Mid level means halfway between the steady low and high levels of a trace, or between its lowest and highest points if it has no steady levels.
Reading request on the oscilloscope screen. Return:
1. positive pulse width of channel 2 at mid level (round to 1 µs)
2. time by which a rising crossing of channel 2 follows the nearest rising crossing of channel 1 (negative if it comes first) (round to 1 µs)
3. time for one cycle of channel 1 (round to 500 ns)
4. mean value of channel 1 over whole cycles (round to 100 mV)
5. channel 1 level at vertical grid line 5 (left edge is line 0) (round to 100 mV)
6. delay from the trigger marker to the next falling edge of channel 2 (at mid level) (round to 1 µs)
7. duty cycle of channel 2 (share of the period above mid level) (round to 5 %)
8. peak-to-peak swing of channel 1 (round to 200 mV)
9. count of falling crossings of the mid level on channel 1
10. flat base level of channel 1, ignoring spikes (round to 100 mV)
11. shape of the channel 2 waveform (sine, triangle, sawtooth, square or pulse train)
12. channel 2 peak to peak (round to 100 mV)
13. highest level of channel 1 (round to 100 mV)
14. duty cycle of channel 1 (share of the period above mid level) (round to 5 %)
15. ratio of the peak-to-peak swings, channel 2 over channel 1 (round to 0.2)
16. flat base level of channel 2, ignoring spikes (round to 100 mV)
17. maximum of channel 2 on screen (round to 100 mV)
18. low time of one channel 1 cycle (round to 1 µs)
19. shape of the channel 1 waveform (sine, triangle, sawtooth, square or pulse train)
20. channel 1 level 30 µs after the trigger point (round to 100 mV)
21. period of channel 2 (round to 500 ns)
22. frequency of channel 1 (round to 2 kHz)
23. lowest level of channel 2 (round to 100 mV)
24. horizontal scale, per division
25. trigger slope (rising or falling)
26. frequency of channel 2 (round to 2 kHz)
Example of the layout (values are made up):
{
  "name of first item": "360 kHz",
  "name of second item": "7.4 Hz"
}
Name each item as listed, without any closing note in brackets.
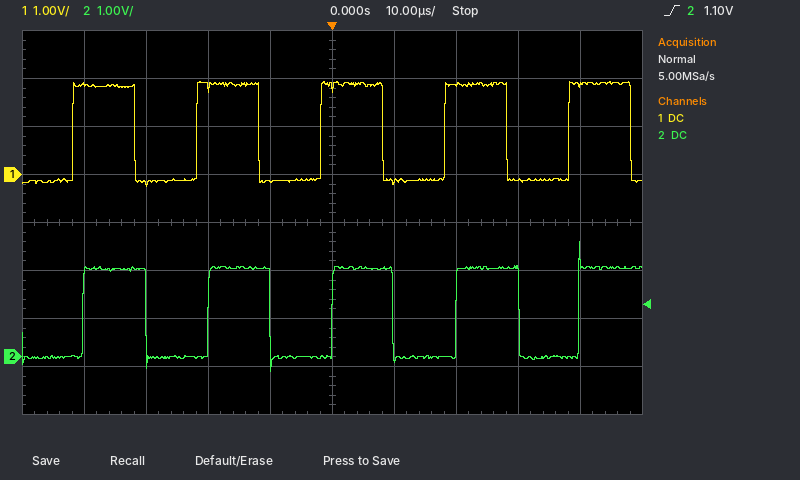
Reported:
{
  "positive pulse width of channel 2 at mid level": "10 µs",
  "time by which a rising crossing of channel 2 follows the nearest rising crossing of channel 1 (negative if it comes first)": "+2 µs",
  "time for one cycle of channel 1": "20.0 µs",
  "mean value of channel 1 over whole cycles": "900 mV",
  "channel 1 level at vertical grid line 5 (left edge is line 0)": "1.8 V",
  "delay from the trigger marker to the next falling edge of channel 2 (at mid level)": "10 µs",
  "duty cycle of channel 2 (share of the period above mid level)": "50 %",
  "peak-to-peak swing of channel 1": "2.2 V",
  "count of falling crossings of the mid level on channel 1": "5",
  "flat base level of channel 1, ignoring spikes": "-100 mV",
  "shape of the channel 2 waveform": "square",
  "channel 2 peak to peak": "2.7 V",
  "highest level of channel 1": "1.9 V",
  "duty cycle of channel 1 (share of the period above mid level)": "50 %",
  "ratio of the peak-to-peak swings, channel 2 over channel 1": "1.2",
  "flat base level of channel 2, ignoring spikes": "0.0 V",
  "maximum of channel 2 on screen": "2.4 V",
  "low time of one channel 1 cycle": "10 µs",
  "shape of the channel 1 waveform": "square",
  "channel 1 level 30 µs after the trigger point": "-100 mV",
  "period of channel 2": "20.0 µs",
  "frequency of channel 1": "50 kHz",
  "lowest level of channel 2": "-300 mV",
  "horizontal scale, per division": "10 µs",
  "trigger slope": "rising",
  "frequency of channel 2": "50 kHz"
}
